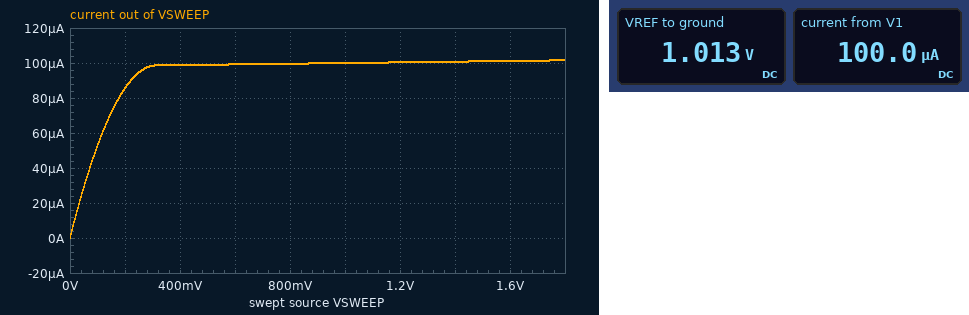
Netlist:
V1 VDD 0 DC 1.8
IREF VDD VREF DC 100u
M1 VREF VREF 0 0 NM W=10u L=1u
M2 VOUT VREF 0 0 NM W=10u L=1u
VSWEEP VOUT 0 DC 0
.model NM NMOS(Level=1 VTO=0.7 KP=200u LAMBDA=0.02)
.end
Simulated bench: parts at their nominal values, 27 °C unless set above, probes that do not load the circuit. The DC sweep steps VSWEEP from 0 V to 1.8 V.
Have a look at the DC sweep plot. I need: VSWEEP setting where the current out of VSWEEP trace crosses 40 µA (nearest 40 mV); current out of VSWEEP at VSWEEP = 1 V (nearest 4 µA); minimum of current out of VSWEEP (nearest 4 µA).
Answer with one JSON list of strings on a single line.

["80 mV", "100 µA", "0 A"]
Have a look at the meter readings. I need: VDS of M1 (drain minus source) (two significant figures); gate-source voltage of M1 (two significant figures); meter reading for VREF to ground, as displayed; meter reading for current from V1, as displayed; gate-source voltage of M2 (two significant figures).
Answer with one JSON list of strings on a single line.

["1.0 V", "1.0 V", "1.013 V", "100.0 µA", "1.0 V"]
